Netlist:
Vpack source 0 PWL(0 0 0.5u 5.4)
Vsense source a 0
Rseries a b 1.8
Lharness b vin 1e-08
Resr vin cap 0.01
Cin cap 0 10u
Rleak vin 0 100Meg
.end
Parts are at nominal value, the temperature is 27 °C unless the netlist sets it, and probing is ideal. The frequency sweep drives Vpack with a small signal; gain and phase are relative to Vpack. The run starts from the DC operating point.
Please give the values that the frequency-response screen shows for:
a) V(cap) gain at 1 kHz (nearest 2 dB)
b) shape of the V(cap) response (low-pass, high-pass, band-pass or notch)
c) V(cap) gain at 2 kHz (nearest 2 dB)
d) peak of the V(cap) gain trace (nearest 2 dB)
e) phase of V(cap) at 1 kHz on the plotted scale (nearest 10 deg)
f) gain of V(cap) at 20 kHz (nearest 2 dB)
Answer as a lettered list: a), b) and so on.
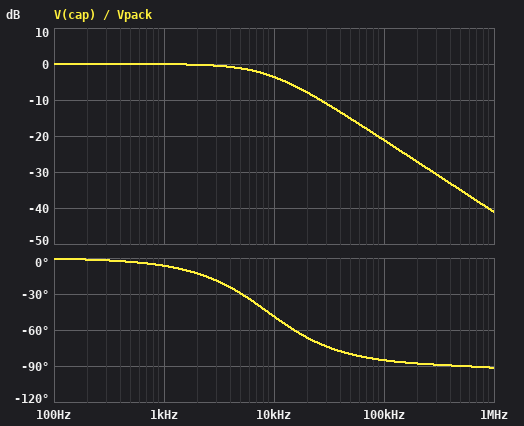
a) 0 dB
b) low-pass
c) 0 dB
d) 0 dB
e) -10 deg
f) -8 dB
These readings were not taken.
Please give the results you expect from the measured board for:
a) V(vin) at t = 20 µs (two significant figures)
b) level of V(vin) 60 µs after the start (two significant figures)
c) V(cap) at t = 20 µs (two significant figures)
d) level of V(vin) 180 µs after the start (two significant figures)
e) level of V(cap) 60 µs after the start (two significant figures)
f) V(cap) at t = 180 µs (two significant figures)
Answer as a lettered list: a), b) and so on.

a) 3.6 V
b) 5.2 V
c) 3.6 V
d) 5.4 V
e) 5.2 V
f) 5.4 V
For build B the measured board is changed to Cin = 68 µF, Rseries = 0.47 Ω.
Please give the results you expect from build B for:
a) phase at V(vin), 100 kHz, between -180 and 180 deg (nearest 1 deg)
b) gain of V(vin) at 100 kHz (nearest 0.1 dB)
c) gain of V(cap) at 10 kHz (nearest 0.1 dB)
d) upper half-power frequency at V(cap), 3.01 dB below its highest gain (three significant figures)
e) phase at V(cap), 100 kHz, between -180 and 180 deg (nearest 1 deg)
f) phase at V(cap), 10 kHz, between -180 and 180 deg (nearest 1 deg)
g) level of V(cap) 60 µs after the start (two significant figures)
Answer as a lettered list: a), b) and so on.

a) -65 deg
b) -25.5 dB
c) -7.2 dB
d) 4.88 kHz
e) -88 deg
f) -64 deg
g) 4.5 V
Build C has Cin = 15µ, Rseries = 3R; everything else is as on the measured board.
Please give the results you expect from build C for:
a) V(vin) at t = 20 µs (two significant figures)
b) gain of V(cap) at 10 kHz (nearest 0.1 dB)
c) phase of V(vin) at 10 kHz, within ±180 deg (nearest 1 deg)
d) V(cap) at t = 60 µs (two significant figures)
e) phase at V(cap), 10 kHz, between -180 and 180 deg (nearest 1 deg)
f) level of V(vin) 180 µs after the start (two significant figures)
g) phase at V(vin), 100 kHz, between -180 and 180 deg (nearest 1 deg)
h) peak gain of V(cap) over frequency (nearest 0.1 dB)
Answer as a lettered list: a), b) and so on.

a) 1.9 V
b) -9.6 dB
c) -70 deg
d) 4.0 V
e) -71 deg
f) 5.3 V
g) -83 deg
h) 0 dB
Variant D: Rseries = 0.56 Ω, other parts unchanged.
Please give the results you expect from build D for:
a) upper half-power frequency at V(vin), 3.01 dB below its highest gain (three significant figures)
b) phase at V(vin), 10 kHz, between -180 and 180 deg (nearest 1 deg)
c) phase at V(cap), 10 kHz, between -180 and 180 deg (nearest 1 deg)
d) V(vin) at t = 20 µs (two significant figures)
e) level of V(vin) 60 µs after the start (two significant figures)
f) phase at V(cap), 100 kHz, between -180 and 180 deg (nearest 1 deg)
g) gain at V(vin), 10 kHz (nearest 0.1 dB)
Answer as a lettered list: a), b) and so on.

a) 28.0 kHz
b) -19 deg
c) -20 deg
d) 5.2 V
e) 5.4 V
f) -75 deg
g) -0.5 dB
